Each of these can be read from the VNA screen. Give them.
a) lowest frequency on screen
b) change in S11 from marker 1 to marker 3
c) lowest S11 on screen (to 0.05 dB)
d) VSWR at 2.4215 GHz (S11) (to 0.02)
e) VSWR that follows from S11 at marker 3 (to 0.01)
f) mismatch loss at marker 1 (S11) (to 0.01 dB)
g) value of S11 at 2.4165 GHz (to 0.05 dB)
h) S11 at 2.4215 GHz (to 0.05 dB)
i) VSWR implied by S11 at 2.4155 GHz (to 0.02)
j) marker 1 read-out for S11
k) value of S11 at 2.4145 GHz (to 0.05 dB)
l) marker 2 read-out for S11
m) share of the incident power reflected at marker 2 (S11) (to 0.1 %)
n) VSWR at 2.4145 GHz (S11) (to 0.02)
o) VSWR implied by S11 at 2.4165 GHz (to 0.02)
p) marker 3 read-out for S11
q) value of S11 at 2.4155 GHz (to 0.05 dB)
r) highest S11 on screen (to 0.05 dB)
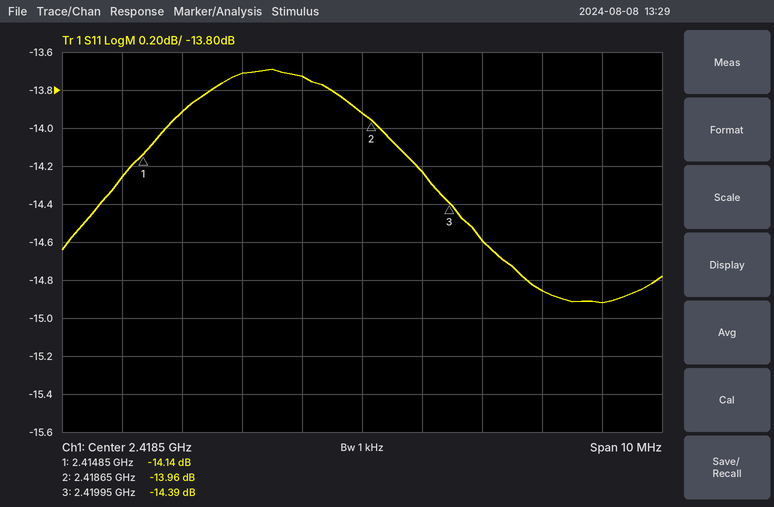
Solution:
2.4135 GHz
-0.25 dB
-14.90 dB
1.44
1.47
0.17 dB
-13.70 dB
-14.85 dB
1.50
-14.14 dB
-14.25 dB
-13.96 dB
4.0 %
1.48
1.52
-14.39 dB
-13.90 dB
-13.70 dB
